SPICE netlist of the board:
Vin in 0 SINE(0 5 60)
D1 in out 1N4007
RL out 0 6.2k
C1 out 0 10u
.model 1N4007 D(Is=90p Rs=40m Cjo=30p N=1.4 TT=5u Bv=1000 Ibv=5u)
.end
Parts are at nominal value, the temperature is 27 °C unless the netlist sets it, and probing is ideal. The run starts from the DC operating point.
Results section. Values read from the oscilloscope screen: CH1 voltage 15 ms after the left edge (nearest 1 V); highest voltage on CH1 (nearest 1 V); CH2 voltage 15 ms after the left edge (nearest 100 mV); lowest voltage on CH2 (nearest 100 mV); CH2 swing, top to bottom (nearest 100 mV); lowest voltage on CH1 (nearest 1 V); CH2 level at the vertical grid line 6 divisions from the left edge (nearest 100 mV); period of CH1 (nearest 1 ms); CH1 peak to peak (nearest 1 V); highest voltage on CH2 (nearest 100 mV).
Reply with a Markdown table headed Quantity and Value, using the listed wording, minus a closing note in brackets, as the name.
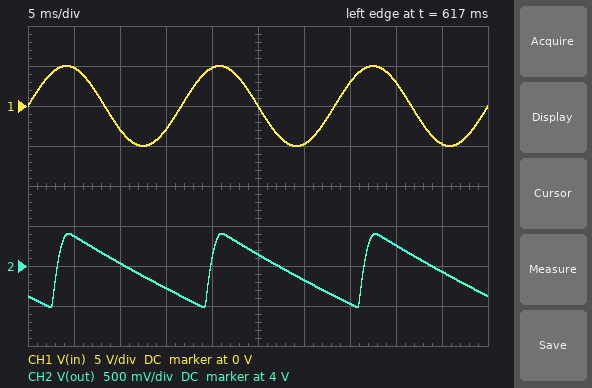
| Quantity | Value |
|---|---|
| CH1 voltage 15 ms after the left edge | -3 V |
| highest voltage on CH1 | 5 V |
| CH2 voltage 15 ms after the left edge | 3.7 V |
| lowest voltage on CH2 | 3.5 V |
| CH2 swing, top to bottom | 900 mV |
| lowest voltage on CH1 | -5 V |
| CH2 level at the vertical grid line 6 divisions from the left edge | 3.8 V |
| period of CH1 | 17 ms |
| CH1 peak to peak | 10 V |
| highest voltage on CH2 | 4.4 V |
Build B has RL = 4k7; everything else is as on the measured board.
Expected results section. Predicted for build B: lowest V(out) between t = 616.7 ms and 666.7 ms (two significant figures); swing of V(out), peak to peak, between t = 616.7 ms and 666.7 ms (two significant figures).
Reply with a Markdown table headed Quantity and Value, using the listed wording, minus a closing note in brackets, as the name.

| Quantity | Value |
|---|---|
| lowest V(out) between t = 616.7 ms and 666.7 ms | 3.2 V |
| swing of V(out), peak to peak, between t = 616.7 ms and 666.7 ms | 1.2 V |
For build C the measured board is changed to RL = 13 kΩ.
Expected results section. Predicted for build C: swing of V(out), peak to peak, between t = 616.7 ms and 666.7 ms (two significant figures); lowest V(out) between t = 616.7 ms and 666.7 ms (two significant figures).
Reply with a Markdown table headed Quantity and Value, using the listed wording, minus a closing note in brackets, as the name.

| Quantity | Value |
|---|---|
| swing of V(out), peak to peak, between t = 616.7 ms and 666.7 ms | 480 mV |
| lowest V(out) between t = 616.7 ms and 666.7 ms | 3.9 V |
